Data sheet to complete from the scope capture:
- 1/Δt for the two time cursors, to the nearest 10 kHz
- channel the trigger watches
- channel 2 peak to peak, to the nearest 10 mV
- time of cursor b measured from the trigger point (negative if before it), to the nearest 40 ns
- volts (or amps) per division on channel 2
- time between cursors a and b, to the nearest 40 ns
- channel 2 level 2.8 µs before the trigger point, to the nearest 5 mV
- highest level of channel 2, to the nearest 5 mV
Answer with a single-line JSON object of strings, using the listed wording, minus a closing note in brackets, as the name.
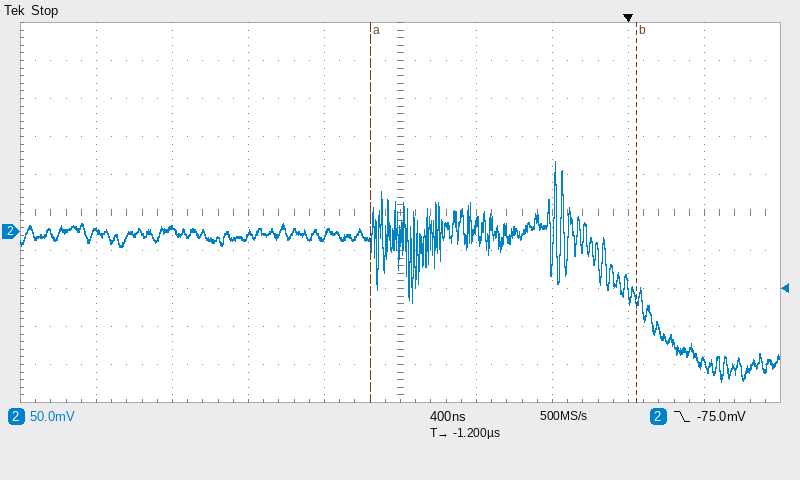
{"1/Δt for the two time cursors, to the nearest 10 kHz": "710 kHz", "channel the trigger watches": "channel 2", "channel 2 peak to peak, to the nearest 10 mV": "290 mV", "time of cursor b measured from the trigger point (negative if before it), to the nearest 40 ns": "+40 ns", "volts (or amps) per division on channel 2": "50 mV", "time between cursors a and b, to the nearest 40 ns": "1.40 µs", "channel 2 level 2.8 µs before the trigger point, to the nearest 5 mV": "0 mV", "highest level of channel 2, to the nearest 5 mV": "90 mV"}
